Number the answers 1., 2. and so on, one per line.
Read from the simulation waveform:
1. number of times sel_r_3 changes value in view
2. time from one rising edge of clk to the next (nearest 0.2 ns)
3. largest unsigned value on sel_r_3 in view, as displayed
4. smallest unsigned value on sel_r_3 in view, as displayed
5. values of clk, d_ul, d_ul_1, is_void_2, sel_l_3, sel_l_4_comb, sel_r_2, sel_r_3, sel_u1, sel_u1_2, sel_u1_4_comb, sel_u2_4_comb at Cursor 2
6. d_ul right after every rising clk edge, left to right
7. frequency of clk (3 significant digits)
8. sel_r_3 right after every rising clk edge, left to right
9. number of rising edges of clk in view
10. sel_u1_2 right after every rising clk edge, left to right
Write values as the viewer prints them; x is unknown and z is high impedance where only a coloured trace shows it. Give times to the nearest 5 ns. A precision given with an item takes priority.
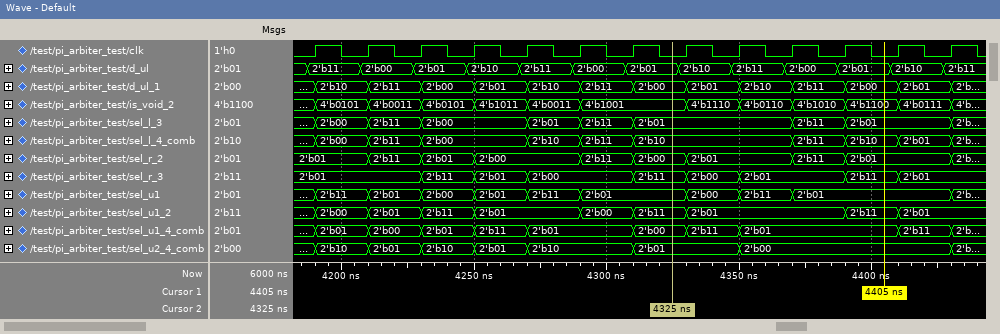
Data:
1. 8
2. 20 ns
3. 2'b11
4. 2'b00
5. clk=0, d_ul=2'b01, d_ul_1=2'b00, is_void_2=4'b1001, sel_l_3=2'b01, sel_l_4_comb=2'b10, sel_r_2=2'b00, sel_r_3=2'b11, sel_u1=2'b01, sel_u1_2=2'b11, sel_u1_4_comb=2'b00, sel_u2_4_comb=2'b01
6. 2'b11, 2'b00, 2'b01, 2'b10, 2'b11, 2'b00, 2'b01, 2'b10, 2'b11, 2'b00, 2'b01, 2'b10, 2'b11
7. 50.0 MHz
8. 2'b01, 2'b01, 2'b11, 2'b01, 2'b00, 2'b00, 2'b11, 2'b00, 2'b01, 2'b01, 2'b11, 2'b01, 2'b01
9. 13
10. 2'b00, 2'b01, 2'b11, 2'b01, 2'b01, 2'b00, 2'b11, 2'b01, 2'b01, 2'b01, 2'b11, 2'b01, 2'b01
